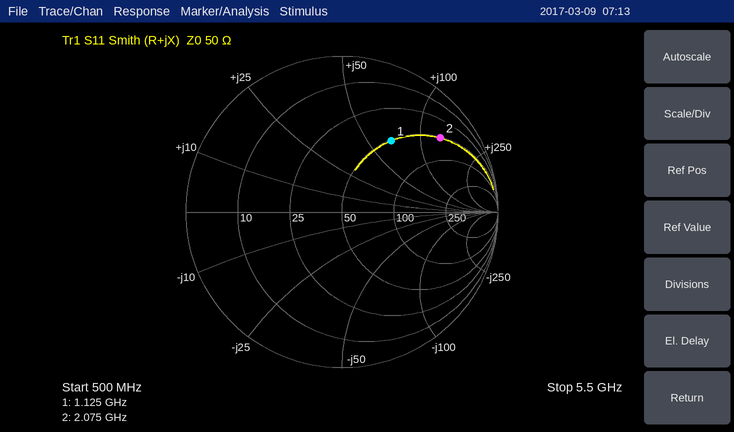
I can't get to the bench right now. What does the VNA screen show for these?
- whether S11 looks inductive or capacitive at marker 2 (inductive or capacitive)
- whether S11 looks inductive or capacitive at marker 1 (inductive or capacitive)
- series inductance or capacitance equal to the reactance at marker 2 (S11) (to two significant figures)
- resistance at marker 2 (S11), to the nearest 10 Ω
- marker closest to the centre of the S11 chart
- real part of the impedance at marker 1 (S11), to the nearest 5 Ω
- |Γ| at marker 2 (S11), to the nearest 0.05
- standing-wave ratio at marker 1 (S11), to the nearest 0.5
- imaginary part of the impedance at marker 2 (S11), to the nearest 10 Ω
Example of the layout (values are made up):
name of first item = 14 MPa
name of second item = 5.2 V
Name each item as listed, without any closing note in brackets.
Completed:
whether S11 looks inductive or capacitive at marker 2 = inductive
whether S11 looks inductive or capacitive at marker 1 = inductive
series inductance or capacitance equal to the reactance at marker 2 (S11) = 10 nH
resistance at marker 2 (S11), to the nearest 10 Ω = 50 Ω
marker closest to the centre of the S11 chart = marker 1
real part of the impedance at marker 1 (S11), to the nearest 5 Ω = 50 Ω
|Γ| at marker 2 (S11), to the nearest 0.05 = 0.80
standing-wave ratio at marker 1 (S11), to the nearest 0.5 = 3.5
imaginary part of the impedance at marker 2 (S11), to the nearest 10 Ω = +130 Ω
